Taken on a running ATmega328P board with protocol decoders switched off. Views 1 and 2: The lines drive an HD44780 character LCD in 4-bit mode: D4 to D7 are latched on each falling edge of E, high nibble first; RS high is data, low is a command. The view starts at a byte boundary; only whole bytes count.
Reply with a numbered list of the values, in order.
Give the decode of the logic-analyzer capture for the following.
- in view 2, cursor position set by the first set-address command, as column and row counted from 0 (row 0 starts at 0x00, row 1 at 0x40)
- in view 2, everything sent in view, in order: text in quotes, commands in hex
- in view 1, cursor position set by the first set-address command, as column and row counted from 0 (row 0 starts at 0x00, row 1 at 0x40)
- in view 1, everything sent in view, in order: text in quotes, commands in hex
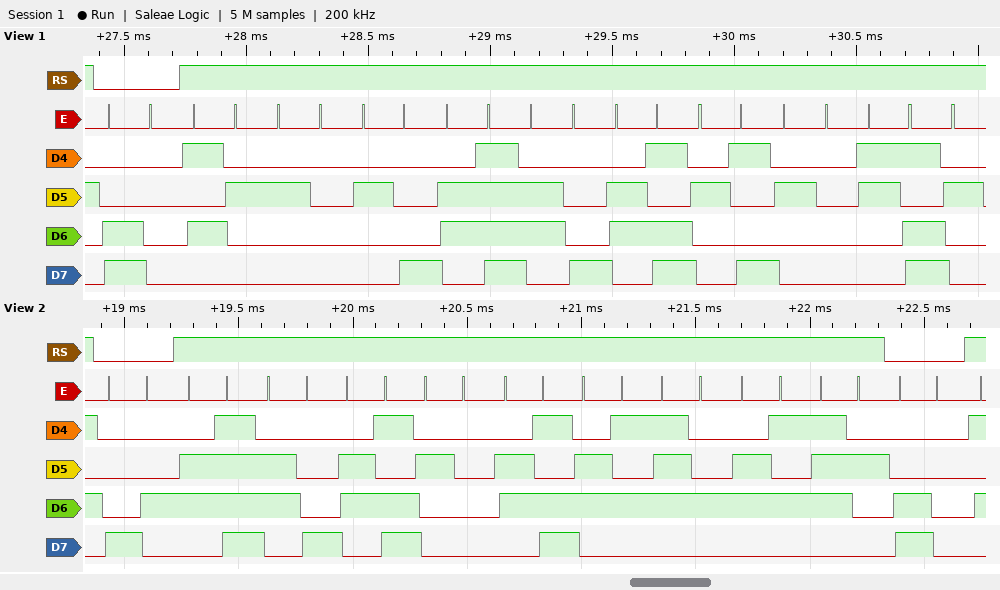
1. column 4, row 0
2. 0x84 "ohm meter" 0xC0
3. column 0, row 1
4. 0xC0 "R (ohm) ="
